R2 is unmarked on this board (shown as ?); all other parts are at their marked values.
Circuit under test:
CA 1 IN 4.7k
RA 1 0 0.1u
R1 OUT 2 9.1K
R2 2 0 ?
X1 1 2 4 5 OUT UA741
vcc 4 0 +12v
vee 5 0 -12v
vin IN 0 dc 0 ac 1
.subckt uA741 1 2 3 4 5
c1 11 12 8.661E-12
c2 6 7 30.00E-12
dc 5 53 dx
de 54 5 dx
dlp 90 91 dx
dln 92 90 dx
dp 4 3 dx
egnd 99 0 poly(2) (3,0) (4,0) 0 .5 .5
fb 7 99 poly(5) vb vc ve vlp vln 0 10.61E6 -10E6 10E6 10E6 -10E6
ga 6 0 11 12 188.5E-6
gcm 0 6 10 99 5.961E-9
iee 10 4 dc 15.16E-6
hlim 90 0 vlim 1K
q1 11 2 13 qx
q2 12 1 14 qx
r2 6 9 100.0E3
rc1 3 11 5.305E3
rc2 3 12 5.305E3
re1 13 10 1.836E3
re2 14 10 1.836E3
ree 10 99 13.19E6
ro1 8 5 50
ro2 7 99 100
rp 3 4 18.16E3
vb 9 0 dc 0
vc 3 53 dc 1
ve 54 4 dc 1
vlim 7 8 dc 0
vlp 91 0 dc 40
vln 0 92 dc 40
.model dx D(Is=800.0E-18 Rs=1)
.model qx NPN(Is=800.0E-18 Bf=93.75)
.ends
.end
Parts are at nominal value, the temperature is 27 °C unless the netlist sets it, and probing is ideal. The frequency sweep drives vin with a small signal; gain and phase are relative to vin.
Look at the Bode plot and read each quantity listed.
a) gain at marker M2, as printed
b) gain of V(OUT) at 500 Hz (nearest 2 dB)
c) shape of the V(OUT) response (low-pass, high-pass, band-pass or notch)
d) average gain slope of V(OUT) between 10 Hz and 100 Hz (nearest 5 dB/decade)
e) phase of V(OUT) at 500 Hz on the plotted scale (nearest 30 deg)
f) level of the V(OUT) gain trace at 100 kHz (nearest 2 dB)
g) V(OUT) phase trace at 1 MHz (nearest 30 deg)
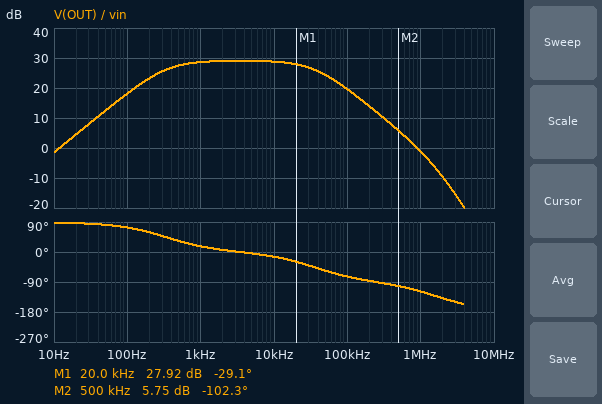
5.75 dB
28 dB
band-pass
20 dB/decade
30 deg
20 dB
-120 deg
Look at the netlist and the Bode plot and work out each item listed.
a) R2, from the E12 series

330 Ω
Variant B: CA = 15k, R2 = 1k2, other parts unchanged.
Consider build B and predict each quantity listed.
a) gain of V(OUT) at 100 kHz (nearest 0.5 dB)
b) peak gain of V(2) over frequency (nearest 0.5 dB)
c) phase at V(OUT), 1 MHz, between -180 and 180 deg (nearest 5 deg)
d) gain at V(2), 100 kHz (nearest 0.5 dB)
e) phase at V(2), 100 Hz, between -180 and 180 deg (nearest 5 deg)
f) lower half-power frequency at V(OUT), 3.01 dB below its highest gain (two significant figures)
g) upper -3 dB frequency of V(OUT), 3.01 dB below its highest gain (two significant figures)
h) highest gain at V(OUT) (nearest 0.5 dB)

16.5 dB
0 dB
-115 deg
-2.0 dB
45 deg
110 Hz
120 kHz
18.5 dB
